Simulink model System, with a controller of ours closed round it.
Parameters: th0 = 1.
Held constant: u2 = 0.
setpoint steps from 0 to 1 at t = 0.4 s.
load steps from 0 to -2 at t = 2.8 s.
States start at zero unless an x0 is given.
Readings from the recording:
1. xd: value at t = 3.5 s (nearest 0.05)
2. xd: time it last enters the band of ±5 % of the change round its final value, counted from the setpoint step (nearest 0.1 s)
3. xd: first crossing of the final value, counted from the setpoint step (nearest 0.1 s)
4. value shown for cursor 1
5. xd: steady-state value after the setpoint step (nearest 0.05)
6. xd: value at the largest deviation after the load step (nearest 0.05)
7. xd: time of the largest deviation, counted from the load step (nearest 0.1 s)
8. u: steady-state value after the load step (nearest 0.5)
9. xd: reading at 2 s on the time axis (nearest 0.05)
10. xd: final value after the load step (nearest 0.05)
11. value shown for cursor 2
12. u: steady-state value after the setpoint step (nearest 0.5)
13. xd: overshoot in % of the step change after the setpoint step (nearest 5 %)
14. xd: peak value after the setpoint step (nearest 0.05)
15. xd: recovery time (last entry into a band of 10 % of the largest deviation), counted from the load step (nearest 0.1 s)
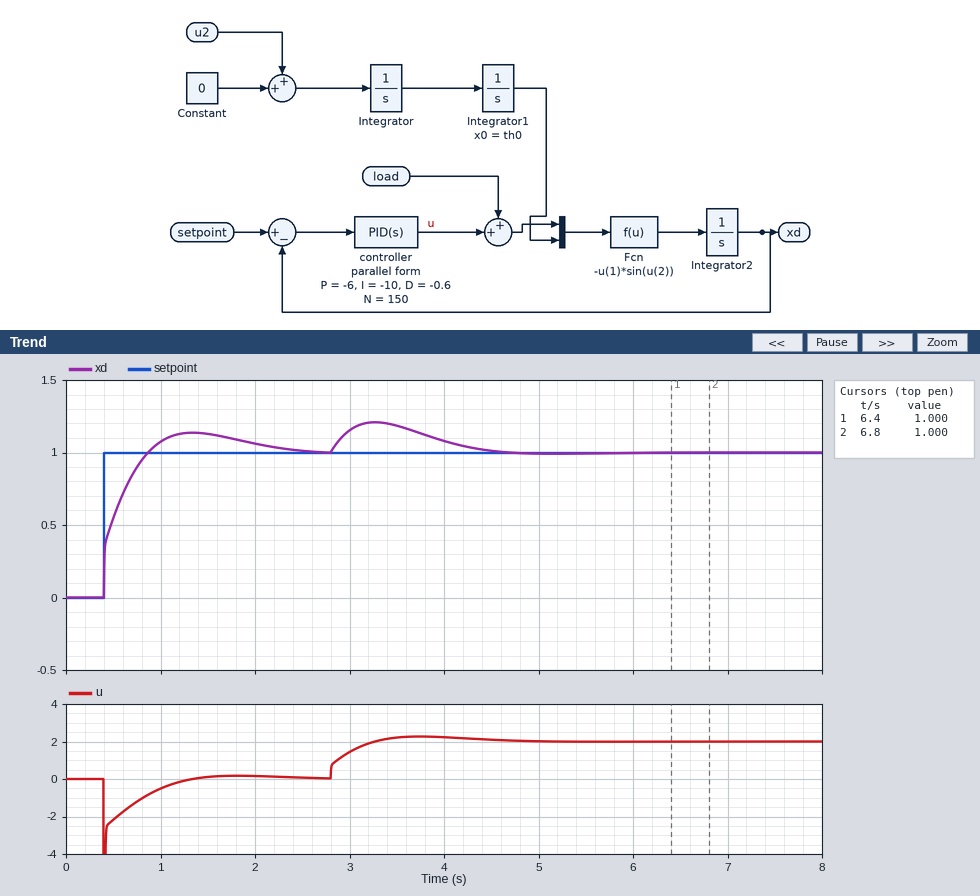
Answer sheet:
1.20
1.7 s
0.5 s
1.000
1.00
1.20
0.5 s
2.0
1.05
1.00
1.000
0.0
15 %
1.15
1.6 s
